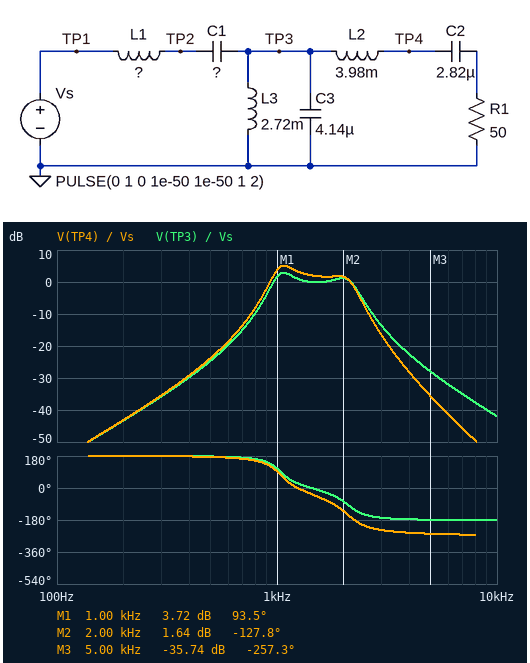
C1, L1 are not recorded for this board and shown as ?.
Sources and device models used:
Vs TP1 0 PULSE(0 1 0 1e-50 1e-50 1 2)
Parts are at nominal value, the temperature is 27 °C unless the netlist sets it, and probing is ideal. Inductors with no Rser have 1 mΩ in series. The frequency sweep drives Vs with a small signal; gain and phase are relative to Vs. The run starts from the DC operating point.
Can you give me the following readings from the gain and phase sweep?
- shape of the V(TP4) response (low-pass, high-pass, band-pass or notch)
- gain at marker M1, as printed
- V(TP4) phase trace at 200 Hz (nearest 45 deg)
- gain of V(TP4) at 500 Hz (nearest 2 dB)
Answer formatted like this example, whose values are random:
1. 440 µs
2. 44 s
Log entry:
1. band-pass
2. 3.72 dB
3. 180 deg
4. -24 dB
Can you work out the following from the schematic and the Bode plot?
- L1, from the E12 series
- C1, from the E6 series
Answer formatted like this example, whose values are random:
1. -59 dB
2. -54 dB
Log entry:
1. 8.2 mH
2. 1.5 µF
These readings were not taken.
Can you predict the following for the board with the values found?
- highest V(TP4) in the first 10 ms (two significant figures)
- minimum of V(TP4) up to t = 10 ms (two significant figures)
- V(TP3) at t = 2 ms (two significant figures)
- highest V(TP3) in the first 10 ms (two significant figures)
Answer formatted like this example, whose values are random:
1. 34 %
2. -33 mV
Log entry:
1. 280 mV
2. -440 mV
3. 51 mV
4. 240 mV
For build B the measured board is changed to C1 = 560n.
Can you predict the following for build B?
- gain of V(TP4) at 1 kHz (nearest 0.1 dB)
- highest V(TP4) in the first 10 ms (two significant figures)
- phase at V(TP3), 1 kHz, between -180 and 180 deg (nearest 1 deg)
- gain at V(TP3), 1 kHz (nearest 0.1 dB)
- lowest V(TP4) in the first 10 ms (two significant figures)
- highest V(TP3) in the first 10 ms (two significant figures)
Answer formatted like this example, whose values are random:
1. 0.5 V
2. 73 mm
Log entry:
1. -12.8 dB
2. 160 mV
3. 143 deg
4. -14.9 dB
5. -250 mV
6. 170 mV
